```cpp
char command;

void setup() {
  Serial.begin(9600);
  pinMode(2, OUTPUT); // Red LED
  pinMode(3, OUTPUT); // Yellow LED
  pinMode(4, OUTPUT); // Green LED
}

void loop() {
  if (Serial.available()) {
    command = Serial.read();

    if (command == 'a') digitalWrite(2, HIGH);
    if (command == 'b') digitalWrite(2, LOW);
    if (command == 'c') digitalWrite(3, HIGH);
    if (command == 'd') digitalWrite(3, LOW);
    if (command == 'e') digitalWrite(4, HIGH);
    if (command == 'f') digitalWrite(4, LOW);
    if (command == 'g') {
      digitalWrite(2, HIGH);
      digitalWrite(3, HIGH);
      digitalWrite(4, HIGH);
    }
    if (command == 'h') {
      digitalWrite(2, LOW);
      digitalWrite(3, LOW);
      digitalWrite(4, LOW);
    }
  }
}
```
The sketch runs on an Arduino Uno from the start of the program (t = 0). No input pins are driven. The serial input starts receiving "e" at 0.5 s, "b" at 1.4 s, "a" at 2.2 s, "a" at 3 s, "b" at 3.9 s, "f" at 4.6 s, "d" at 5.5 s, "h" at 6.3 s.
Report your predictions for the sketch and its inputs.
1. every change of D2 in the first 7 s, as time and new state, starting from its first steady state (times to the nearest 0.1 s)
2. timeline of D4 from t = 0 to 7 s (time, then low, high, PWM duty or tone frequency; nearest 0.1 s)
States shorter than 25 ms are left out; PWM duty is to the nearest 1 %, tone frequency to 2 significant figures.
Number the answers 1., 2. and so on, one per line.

1. 0 s low; 2.2 s high; 3.9 s low
2. 0 s low; 0.5 s high; 4.6 s low
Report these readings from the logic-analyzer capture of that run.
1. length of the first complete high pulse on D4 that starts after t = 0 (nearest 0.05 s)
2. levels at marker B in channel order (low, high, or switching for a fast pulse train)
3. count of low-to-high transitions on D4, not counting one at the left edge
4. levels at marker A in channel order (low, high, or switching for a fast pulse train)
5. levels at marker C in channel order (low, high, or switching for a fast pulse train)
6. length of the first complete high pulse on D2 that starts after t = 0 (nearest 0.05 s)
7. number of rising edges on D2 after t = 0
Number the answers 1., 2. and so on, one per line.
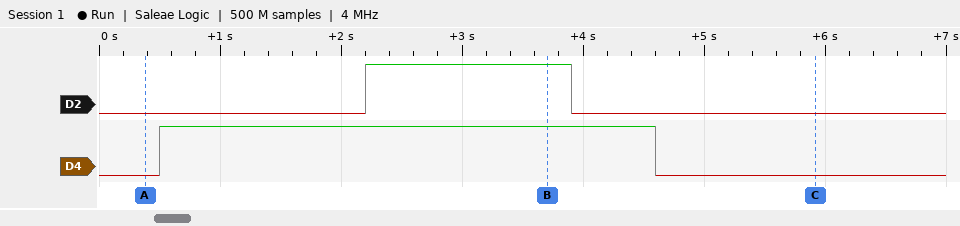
1. 4.10 s
2. D2 high, D4 high
3. 1
4. D2 low, D4 low
5. D2 low, D4 low
6. 1.70 s
7. 1
